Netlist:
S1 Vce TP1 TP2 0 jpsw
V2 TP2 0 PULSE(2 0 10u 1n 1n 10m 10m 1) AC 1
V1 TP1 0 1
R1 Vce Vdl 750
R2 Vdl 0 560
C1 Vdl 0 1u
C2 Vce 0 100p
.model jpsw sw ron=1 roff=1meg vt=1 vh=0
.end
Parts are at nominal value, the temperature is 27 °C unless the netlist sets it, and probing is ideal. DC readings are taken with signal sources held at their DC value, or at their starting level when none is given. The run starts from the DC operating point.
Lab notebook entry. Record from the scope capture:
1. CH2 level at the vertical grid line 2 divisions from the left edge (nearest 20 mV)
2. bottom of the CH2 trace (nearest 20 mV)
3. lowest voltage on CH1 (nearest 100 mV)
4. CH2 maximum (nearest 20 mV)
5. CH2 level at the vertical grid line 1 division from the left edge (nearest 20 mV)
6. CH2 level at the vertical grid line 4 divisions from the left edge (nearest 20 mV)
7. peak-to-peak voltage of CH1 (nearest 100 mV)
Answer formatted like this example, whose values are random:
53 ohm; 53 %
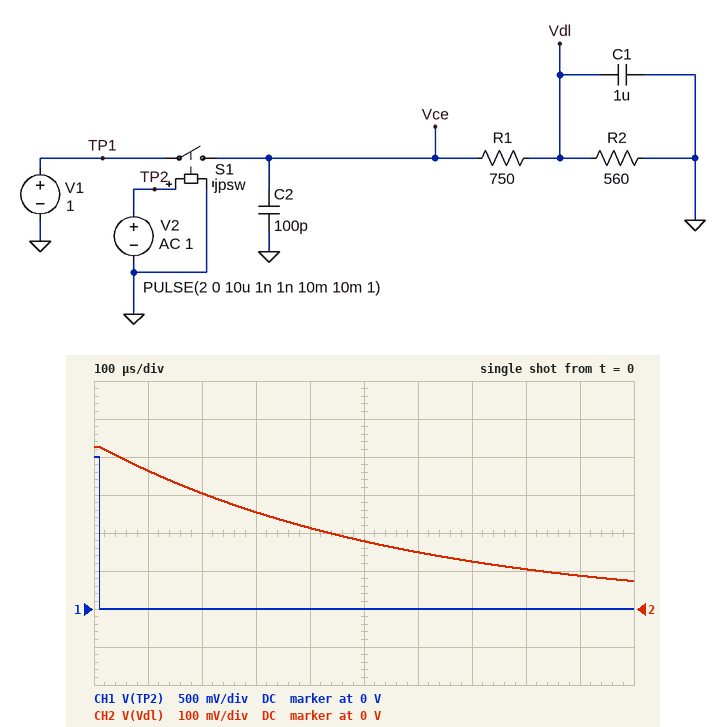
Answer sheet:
300 mV; 80 mV; 0 V; 420 mV; 360 mV; 220 mV; 2.0 V
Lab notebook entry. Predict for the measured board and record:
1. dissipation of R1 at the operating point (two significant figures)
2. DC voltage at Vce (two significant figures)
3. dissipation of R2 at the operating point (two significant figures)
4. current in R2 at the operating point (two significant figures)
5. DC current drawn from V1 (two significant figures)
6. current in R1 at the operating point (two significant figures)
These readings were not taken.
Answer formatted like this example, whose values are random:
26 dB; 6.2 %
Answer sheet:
440 µW; 1.0 V; 330 µW; 760 µA; 760 µA; 760 µA
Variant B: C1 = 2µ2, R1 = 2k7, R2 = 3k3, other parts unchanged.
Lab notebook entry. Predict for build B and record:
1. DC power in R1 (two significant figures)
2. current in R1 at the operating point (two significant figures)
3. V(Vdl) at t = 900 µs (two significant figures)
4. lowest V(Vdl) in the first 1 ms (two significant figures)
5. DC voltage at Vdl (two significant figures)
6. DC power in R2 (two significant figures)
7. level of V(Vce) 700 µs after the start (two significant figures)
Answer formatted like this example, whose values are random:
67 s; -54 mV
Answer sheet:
75 µW; 170 µA; 490 mV; 480 mV; 550 mV; 92 µW; 500 mV
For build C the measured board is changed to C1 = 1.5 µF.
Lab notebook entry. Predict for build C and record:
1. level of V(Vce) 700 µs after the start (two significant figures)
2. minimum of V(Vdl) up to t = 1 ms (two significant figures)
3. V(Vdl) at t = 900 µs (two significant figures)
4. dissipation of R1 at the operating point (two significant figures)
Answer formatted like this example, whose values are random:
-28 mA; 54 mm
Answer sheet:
190 mV; 130 mV; 150 mV; 440 µW
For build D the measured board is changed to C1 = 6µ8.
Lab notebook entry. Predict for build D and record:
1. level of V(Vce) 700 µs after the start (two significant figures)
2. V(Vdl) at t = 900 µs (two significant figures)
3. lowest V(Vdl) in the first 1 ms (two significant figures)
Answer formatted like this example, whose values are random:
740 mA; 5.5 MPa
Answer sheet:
360 mV; 340 mV; 330 mV
